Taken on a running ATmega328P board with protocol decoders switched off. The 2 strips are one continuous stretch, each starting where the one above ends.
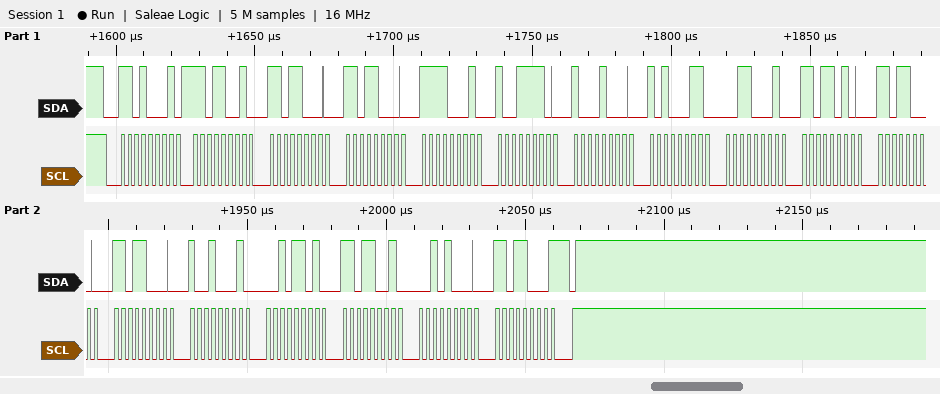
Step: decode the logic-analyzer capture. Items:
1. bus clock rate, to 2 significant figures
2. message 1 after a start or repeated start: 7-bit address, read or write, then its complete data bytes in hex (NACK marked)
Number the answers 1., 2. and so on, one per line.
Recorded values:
1. 400 kHz
2. 0x68 read: D9 D8 D8 F1 9E 88 A3 31 DA D8 D8 91 2D D9 28 D8 NACK
